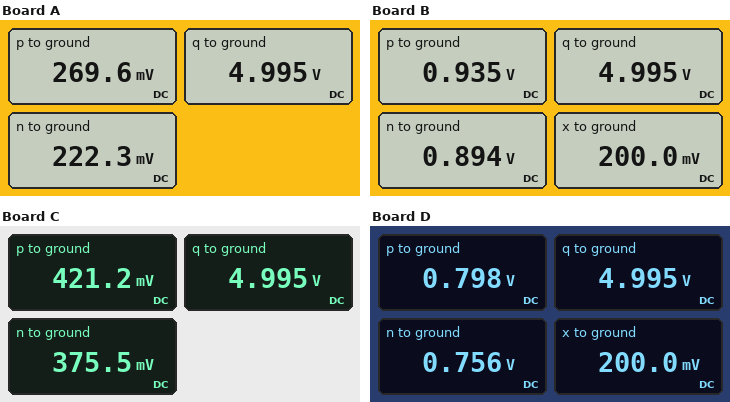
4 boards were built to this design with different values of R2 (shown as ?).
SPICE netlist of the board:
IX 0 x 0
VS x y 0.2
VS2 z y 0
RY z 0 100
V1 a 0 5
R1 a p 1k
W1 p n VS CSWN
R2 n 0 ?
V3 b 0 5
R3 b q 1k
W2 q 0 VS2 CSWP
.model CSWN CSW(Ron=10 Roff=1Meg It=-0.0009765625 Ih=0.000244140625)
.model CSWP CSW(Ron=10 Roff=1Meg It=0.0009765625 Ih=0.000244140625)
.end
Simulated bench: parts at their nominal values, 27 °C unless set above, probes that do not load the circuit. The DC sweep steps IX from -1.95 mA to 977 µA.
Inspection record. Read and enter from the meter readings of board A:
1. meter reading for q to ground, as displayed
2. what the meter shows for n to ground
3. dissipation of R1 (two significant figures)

4.995 V
222.3 mV
22 mW
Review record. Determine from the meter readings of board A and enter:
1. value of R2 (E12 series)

47 Ω
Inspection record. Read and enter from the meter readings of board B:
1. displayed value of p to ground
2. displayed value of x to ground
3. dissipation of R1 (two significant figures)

0.935 V
200.0 mV
17 mW
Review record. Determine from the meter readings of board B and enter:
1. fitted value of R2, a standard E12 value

220 Ω
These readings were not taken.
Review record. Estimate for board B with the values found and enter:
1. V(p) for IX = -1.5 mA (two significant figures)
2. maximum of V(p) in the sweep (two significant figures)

5.0 V
5.0 V
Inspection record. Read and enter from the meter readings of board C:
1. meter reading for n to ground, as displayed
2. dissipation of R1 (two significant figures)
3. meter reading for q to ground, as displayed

375.5 mV
21 mW
4.995 V
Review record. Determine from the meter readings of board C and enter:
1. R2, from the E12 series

82 Ω
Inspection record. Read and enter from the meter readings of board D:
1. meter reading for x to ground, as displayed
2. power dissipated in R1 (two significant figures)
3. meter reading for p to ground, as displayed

200.0 mV
18 mW
0.798 V
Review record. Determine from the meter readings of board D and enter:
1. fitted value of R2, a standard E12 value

180 Ω
